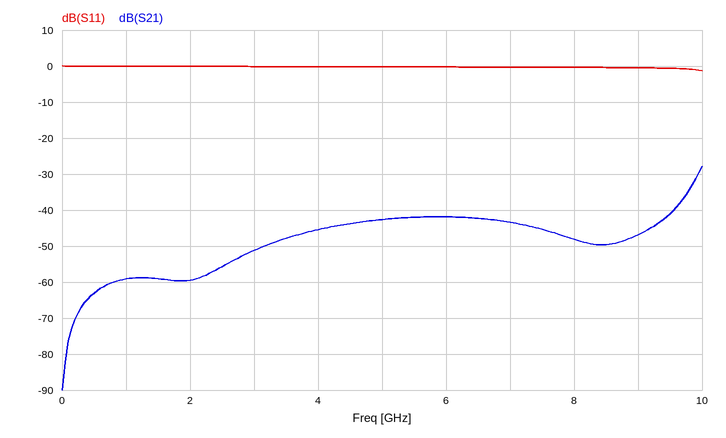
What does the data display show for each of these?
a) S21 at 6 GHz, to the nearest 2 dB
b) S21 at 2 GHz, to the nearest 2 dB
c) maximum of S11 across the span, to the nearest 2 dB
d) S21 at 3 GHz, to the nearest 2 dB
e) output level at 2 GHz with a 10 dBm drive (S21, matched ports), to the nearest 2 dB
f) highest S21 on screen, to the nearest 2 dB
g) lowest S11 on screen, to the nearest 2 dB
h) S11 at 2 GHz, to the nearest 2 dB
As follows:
-42 dB
-60 dB
0 dB
-52 dB
-50 dBm
-28 dB
-2 dB
0 dB
